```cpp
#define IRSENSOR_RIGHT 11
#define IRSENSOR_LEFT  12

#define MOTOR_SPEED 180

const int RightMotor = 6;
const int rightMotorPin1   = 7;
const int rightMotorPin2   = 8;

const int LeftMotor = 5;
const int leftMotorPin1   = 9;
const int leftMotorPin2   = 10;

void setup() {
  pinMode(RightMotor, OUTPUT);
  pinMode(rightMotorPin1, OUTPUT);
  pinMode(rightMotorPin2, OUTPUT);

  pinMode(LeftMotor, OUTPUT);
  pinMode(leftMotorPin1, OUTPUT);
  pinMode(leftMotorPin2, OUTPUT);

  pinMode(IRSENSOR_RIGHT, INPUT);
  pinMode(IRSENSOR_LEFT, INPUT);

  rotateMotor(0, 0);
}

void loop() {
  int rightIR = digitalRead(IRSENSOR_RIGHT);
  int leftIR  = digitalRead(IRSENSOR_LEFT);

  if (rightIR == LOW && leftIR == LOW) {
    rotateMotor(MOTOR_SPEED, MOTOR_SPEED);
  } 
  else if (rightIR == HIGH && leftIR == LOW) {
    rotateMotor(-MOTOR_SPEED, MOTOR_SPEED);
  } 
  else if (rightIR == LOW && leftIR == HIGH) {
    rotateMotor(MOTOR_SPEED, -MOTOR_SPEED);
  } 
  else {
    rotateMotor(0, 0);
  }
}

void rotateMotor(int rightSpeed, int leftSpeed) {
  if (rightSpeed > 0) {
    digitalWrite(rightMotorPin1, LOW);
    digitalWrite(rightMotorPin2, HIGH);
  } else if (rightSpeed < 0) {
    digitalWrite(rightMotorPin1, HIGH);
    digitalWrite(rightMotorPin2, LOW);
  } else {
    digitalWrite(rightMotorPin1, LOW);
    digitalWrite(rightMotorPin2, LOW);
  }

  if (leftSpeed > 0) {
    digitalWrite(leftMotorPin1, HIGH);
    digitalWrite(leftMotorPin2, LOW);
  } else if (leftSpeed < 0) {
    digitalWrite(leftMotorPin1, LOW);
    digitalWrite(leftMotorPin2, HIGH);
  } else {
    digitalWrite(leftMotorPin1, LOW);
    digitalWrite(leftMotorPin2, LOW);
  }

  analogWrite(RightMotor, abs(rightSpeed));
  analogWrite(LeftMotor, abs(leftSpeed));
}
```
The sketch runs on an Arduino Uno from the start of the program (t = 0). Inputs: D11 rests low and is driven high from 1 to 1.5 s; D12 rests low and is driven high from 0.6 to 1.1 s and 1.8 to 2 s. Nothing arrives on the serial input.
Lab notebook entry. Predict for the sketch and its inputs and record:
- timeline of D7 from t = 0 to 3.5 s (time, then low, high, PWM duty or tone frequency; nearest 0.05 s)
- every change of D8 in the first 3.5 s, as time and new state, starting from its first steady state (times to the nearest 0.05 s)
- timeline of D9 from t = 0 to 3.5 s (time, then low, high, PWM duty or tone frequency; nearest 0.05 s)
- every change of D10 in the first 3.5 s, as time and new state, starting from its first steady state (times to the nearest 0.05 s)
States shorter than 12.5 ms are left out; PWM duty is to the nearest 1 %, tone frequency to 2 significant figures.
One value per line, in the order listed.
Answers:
0 s low; 1.1 s high; 1.5 s low
0 s high; 1 s low; 1.5 s high
0 s high; 0.6 s low; 1.1 s high; 1.8 s low; 2 s high
0 s low; 0.6 s high; 1 s low; 1.8 s high; 2 s low
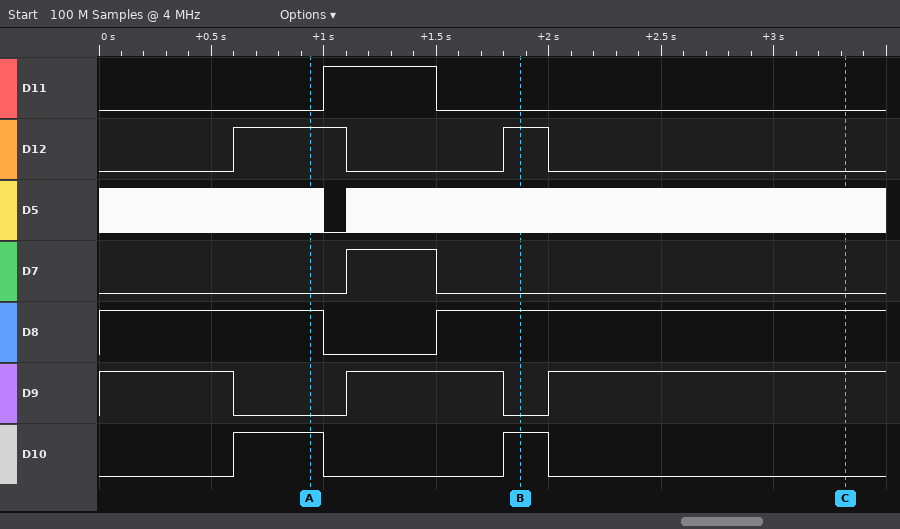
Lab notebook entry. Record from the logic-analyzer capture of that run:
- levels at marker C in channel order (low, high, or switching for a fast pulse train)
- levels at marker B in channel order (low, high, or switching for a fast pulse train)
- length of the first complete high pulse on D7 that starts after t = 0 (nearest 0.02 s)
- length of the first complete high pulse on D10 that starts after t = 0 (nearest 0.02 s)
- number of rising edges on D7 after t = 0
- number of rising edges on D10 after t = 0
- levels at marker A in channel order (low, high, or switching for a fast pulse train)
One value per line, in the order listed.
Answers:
D11 low, D12 low, D5 switching, D7 low, D8 high, D9 high, D10 low
D11 low, D12 high, D5 switching, D7 low, D8 high, D9 low, D10 high
0.40 s
0.40 s
1
2
D11 low, D12 high, D5 switching, D7 low, D8 high, D9 low, D10 high
